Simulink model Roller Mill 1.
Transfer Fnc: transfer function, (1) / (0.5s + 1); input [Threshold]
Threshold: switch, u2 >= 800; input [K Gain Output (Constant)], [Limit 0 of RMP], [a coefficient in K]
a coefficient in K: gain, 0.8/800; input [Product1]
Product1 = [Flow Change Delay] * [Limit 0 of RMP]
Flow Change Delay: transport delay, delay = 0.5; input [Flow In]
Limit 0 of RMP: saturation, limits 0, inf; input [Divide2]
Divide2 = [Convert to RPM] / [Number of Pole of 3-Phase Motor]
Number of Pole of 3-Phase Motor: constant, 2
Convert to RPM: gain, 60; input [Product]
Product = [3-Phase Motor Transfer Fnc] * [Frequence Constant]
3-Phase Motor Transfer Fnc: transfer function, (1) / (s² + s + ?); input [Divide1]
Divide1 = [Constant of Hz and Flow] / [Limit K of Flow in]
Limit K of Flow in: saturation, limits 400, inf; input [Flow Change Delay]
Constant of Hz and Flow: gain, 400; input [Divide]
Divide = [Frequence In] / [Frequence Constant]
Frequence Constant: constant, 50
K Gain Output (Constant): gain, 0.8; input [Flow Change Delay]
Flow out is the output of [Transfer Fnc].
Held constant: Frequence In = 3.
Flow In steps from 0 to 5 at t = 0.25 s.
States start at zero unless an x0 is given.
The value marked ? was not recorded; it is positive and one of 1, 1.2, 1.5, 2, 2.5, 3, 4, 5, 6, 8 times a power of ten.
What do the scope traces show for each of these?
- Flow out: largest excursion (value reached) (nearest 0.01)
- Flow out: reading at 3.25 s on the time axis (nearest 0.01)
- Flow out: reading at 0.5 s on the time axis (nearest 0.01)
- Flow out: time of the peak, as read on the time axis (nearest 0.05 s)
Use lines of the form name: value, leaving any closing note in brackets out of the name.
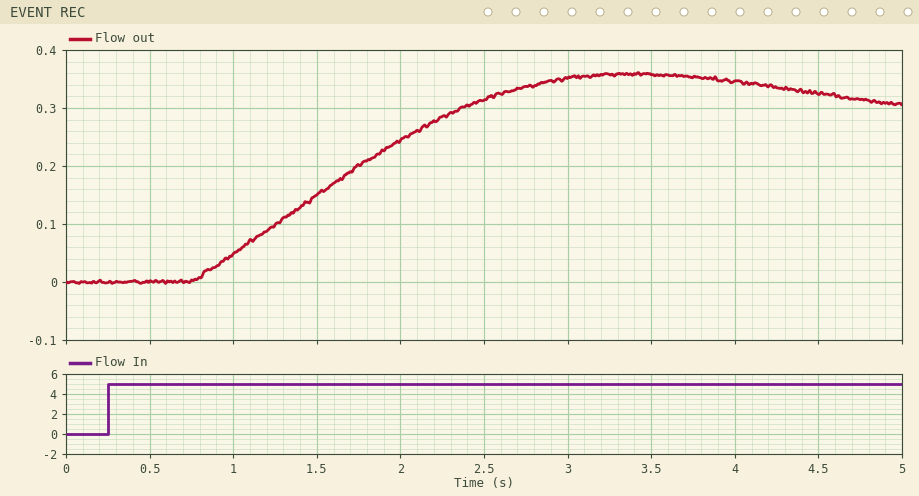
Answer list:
Flow out: largest excursion (value reached): 0.36
Flow out: reading at 3.25 s on the time axis: 0.36
Flow out: reading at 0.5 s on the time axis: 0.00
Flow out: time of the peak, as read on the time axis: 3.40 s
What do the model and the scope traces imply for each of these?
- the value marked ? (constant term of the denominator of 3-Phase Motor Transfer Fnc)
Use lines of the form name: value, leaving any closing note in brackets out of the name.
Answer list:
the value marked ?: 1.5
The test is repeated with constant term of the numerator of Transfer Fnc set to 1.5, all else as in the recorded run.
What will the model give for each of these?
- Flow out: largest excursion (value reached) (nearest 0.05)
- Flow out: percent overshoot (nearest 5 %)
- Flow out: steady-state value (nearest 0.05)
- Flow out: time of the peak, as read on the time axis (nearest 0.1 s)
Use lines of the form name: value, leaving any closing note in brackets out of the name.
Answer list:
Flow out: largest excursion (value reached): 0.55
Flow out: percent overshoot: 20 %
Flow out: steady-state value: 0.45
Flow out: time of the peak, as read on the time axis: 3.4 s
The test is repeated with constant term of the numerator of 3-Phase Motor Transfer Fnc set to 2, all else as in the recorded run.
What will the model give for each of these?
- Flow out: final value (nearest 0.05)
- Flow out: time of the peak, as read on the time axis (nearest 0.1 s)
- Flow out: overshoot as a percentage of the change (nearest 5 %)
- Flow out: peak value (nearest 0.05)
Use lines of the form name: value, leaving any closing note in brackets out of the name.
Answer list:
Flow out: final value: 0.60
Flow out: time of the peak, as read on the time axis: 3.4 s
Flow out: overshoot as a percentage of the change: 20 %
Flow out: peak value: 0.70
